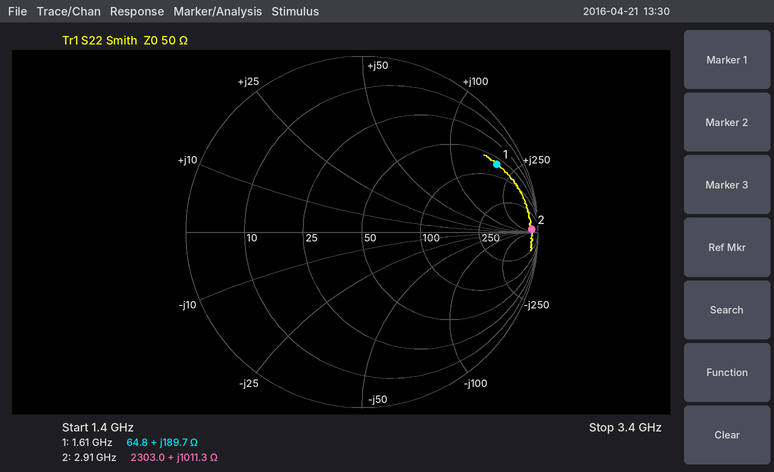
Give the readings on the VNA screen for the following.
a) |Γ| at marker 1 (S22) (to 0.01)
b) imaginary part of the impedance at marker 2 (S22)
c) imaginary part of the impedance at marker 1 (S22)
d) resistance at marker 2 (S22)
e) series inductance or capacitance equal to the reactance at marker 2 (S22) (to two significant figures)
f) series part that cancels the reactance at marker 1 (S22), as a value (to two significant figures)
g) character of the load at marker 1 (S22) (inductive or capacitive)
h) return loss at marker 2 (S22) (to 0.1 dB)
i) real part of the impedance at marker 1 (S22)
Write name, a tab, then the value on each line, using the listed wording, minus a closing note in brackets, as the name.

|Γ| at marker 1 (S22)	0.86
imaginary part of the impedance at marker 2	+1011.3 Ω
imaginary part of the impedance at marker 1	+189.7 Ω
resistance at marker 2	2303.0 Ω
series inductance or capacitance equal to the reactance at marker 2 (S22)	55 nH
series part that cancels the reactance at marker 1 (S22), as a value	520 fF
character of the load at marker 1 (S22)	inductive
return loss at marker 2 (S22)	0.3 dB
real part of the impedance at marker 1	64.8 Ω
